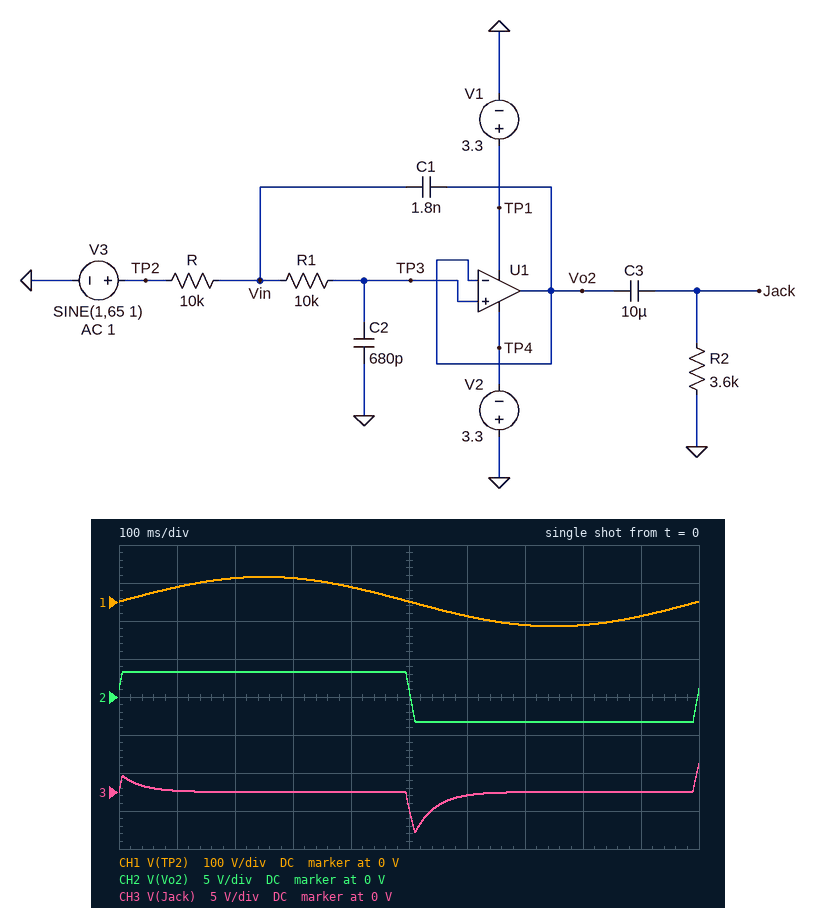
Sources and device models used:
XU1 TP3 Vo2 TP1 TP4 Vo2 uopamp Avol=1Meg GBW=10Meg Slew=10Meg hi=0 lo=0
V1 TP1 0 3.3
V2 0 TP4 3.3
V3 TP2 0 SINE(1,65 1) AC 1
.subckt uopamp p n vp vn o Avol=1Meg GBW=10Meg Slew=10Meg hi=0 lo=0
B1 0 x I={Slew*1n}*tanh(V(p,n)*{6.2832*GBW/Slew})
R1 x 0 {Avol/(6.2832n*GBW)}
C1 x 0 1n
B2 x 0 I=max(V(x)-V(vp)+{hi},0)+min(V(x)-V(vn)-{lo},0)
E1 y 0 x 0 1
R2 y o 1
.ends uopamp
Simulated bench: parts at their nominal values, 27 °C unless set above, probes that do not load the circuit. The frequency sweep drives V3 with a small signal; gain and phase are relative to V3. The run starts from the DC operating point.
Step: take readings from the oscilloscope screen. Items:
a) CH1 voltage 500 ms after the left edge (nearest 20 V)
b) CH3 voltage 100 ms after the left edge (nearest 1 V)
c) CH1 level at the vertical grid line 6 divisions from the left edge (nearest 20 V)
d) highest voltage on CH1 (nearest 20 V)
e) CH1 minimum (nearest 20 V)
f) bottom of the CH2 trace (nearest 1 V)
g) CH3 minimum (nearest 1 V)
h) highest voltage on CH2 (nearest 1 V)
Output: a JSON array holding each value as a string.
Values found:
["0 V", "0 V", "-40 V", "60 V", "-60 V", "-3 V", "-5 V", "3 V"]
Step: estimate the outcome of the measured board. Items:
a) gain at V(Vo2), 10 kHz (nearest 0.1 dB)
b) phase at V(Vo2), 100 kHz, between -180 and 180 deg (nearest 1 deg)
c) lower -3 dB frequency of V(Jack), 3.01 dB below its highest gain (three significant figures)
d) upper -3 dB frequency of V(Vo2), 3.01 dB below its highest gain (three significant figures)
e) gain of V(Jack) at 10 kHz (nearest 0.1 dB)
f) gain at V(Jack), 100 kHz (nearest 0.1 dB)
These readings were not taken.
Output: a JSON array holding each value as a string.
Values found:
["0 dB", "-170 deg", "4.72 Hz", "15.8 kHz", "0 dB", "-33.7 dB"]
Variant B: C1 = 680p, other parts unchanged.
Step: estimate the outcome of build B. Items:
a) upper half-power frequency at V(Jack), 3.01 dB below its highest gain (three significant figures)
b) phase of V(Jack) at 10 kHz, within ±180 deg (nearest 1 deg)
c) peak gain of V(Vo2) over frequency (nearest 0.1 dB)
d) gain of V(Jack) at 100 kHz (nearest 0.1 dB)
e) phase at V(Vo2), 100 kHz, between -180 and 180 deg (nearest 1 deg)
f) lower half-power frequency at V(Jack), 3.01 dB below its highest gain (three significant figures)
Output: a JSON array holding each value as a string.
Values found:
["15.1 kHz", "-46 deg", "0 dB", "-25.7 dB", "-154 deg", "4.42 Hz"]
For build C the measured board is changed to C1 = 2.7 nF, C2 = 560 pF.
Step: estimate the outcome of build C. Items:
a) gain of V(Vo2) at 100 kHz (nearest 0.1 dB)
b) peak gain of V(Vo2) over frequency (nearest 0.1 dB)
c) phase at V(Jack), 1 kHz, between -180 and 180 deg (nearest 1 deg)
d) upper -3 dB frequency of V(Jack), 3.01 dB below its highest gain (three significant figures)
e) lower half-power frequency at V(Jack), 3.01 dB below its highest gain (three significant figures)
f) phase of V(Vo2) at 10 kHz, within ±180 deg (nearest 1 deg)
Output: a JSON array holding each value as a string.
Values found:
["-35.5 dB", "1.8 dB", "-4 deg", "15.3 kHz", "7.91 Hz", "-60 deg"]
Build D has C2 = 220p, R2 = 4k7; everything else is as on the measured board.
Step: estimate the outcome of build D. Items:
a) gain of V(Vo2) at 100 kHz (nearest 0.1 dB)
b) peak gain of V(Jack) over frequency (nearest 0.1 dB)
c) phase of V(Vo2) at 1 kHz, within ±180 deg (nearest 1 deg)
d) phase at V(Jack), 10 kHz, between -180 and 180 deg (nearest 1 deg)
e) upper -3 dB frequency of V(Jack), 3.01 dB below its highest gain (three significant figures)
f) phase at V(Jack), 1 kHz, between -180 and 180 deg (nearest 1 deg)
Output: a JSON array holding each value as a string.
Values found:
["-23.5 dB", "3.7 dB", "-2 deg", "-18 deg", "29.9 kHz", "-1 deg"]
